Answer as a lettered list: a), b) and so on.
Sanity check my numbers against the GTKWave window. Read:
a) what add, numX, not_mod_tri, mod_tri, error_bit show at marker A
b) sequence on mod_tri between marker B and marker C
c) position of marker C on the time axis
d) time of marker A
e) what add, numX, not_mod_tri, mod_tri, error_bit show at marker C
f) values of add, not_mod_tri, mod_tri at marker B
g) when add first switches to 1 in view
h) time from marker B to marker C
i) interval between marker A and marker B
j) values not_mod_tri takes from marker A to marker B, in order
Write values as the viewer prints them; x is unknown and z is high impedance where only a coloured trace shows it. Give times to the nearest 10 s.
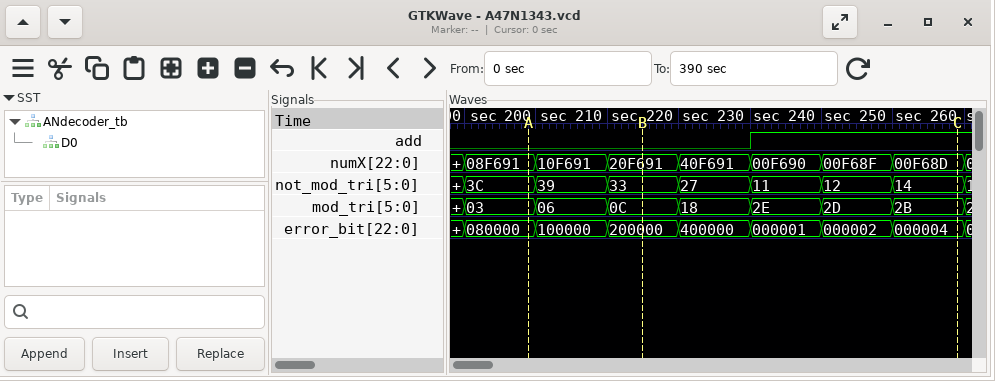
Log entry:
a) add=0, numX=08F691, not_mod_tri=3C, mod_tri=03, error_bit=080000
b) 0C, 18, 2E, 2D, 2B
c) 260 s
d) 200 s
e) add=1, numX=00F68D, not_mod_tri=14, mod_tri=2B, error_bit=000004
f) add=0, not_mod_tri=33, mod_tri=0C
g) 230 s
h) 40 s
i) 20 s
j) 3C, 39, 33
